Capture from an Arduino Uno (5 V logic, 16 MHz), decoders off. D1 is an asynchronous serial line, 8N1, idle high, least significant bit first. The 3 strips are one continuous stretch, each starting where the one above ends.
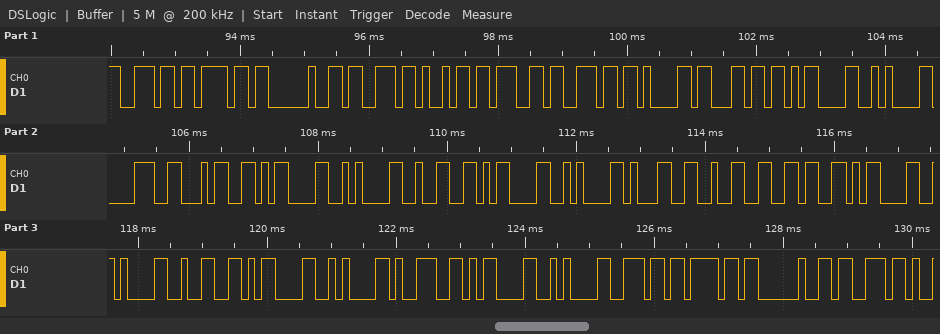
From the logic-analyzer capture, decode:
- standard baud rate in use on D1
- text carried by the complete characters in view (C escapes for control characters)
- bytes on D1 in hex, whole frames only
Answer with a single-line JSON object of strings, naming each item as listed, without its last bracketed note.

{"standard baud rate in use on D1": "9600 baud", "text carried by the complete characters in view": "\"no signal\\r\\n84\\r\\n2\\r\\n126\\r\\n2\\r\\n9\\r\\nno s\"", "bytes on D1 in hex, whole frames only": "6E 6F 20 73 69 67 6E 61 6C 0D 0A 38 34 0D 0A 32 0D 0A 31 32 36 0D 0A 32 0D 0A 39 0D 0A 6E 6F 20 73"}
